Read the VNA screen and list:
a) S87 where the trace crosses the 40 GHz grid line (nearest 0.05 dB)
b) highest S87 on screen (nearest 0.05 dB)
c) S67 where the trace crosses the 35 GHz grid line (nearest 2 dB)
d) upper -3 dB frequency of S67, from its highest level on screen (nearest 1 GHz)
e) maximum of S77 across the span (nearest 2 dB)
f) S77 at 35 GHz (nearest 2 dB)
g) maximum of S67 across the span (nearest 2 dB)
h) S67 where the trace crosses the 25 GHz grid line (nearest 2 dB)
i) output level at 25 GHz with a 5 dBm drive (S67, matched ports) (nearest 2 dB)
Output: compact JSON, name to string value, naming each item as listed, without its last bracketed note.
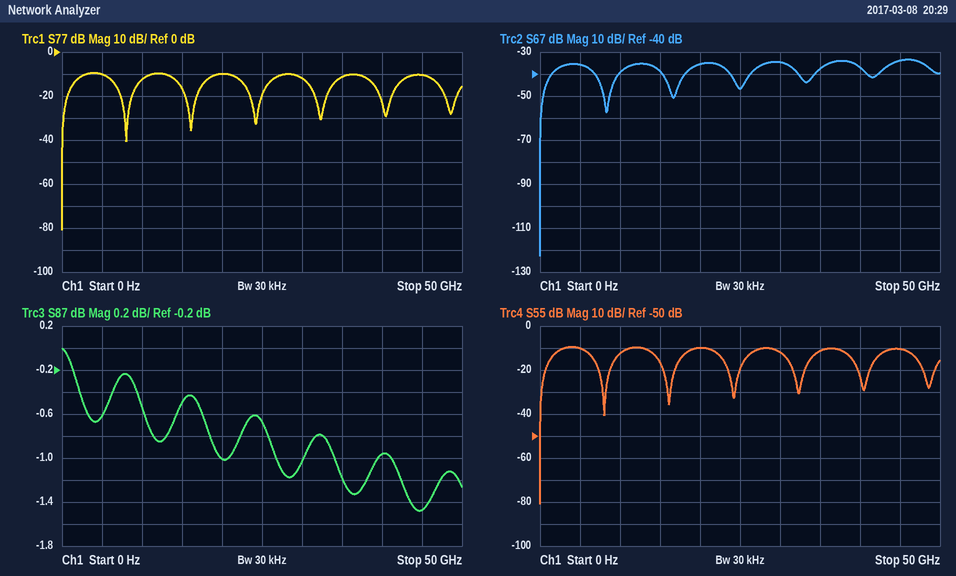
{"S87 where the trace crosses the 40 GHz grid line": "-0.95 dB", "highest S87 on screen": "0.00 dB", "S67 where the trace crosses the 35 GHz grid line": "-38 dB", "upper -3 dB frequency of S67, from its highest level on screen": "48 GHz", "maximum of S77 across the span": "-10 dB", "S77 at 35 GHz": "-12 dB", "maximum of S67 across the span": "-34 dB", "S67 where the trace crosses the 25 GHz grid line": "-46 dB", "output level at 25 GHz with a 5 dBm drive (S67, matched ports)": "-42 dBm"}
